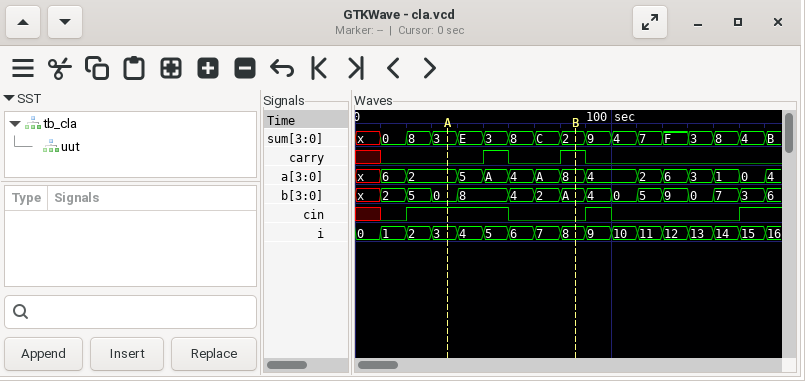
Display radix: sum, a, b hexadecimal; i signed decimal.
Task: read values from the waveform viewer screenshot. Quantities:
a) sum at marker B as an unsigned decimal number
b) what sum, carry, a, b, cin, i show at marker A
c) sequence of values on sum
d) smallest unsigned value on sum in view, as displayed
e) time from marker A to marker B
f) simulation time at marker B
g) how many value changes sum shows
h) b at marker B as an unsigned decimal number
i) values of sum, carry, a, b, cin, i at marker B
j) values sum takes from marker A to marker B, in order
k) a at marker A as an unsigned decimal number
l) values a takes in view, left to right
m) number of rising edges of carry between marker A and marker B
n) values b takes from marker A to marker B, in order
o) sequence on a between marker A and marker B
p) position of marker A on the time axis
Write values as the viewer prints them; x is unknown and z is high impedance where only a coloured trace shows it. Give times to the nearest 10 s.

2
sum=3, carry=0, a=2, b=0, cin=1, i=3
x, 0, 8, 3, E, 3, 8, C, 2, 9, 4, 7, F, 3, 8, 4, B
0
50 s
90 s
16
10
sum=2, carry=1, a=8, b=A, cin=0, i=8
3, E, 3, 8, C, 2
2
x, 6, 2, 5, A, 4, A, 8, 4, 2, 6, 3, 1, 0, 4
2
0, 8, 4, 2, A
2, 5, A, 4, A, 8
40 s
